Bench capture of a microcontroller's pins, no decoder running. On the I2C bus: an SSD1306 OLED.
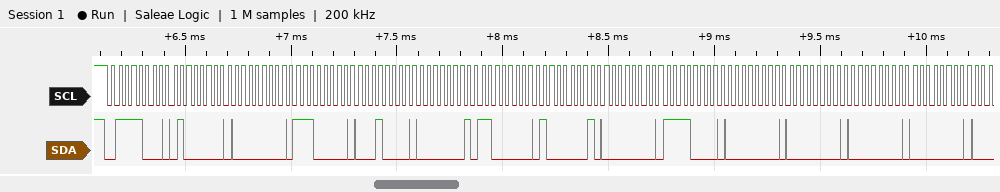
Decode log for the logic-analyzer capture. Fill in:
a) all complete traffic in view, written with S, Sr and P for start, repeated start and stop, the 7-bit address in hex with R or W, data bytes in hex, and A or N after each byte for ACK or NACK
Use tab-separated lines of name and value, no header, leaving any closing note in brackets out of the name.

all complete traffic in view, written with S, Sr and P for start, repeated start and stop, the 7-bit address in hex with R or W, data bytes in hex, and A or N after each byte for ACK or NACK	S 3CW A 40 A 00 A E0 A 10 A 01 A C0 A 81 A 00 A F0 A 00 A 00 A 00 A 00 A
